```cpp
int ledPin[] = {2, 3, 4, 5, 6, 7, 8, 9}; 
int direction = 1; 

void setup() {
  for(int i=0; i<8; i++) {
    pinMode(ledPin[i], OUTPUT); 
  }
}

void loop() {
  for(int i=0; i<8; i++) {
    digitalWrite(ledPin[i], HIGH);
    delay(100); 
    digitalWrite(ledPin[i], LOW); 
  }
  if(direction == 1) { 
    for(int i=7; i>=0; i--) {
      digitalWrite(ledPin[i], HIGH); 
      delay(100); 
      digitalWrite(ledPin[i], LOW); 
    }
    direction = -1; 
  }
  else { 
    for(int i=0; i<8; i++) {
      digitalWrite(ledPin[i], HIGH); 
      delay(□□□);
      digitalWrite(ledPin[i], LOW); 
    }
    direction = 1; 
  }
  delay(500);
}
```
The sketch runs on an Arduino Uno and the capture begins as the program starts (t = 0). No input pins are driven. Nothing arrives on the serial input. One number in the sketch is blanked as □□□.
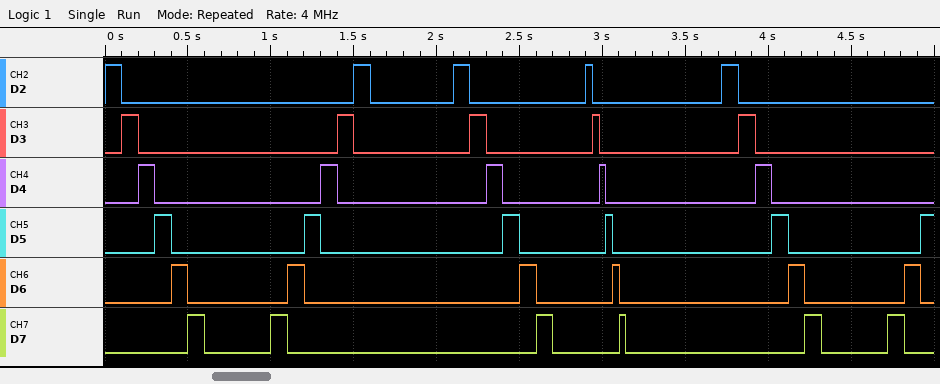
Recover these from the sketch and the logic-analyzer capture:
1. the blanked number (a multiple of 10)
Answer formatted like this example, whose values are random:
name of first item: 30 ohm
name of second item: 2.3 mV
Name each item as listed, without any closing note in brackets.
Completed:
the blanked number: 40
